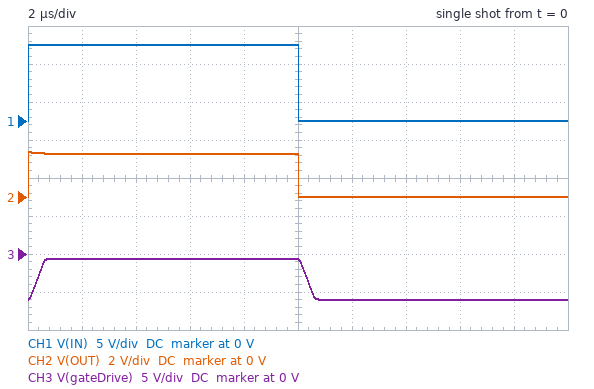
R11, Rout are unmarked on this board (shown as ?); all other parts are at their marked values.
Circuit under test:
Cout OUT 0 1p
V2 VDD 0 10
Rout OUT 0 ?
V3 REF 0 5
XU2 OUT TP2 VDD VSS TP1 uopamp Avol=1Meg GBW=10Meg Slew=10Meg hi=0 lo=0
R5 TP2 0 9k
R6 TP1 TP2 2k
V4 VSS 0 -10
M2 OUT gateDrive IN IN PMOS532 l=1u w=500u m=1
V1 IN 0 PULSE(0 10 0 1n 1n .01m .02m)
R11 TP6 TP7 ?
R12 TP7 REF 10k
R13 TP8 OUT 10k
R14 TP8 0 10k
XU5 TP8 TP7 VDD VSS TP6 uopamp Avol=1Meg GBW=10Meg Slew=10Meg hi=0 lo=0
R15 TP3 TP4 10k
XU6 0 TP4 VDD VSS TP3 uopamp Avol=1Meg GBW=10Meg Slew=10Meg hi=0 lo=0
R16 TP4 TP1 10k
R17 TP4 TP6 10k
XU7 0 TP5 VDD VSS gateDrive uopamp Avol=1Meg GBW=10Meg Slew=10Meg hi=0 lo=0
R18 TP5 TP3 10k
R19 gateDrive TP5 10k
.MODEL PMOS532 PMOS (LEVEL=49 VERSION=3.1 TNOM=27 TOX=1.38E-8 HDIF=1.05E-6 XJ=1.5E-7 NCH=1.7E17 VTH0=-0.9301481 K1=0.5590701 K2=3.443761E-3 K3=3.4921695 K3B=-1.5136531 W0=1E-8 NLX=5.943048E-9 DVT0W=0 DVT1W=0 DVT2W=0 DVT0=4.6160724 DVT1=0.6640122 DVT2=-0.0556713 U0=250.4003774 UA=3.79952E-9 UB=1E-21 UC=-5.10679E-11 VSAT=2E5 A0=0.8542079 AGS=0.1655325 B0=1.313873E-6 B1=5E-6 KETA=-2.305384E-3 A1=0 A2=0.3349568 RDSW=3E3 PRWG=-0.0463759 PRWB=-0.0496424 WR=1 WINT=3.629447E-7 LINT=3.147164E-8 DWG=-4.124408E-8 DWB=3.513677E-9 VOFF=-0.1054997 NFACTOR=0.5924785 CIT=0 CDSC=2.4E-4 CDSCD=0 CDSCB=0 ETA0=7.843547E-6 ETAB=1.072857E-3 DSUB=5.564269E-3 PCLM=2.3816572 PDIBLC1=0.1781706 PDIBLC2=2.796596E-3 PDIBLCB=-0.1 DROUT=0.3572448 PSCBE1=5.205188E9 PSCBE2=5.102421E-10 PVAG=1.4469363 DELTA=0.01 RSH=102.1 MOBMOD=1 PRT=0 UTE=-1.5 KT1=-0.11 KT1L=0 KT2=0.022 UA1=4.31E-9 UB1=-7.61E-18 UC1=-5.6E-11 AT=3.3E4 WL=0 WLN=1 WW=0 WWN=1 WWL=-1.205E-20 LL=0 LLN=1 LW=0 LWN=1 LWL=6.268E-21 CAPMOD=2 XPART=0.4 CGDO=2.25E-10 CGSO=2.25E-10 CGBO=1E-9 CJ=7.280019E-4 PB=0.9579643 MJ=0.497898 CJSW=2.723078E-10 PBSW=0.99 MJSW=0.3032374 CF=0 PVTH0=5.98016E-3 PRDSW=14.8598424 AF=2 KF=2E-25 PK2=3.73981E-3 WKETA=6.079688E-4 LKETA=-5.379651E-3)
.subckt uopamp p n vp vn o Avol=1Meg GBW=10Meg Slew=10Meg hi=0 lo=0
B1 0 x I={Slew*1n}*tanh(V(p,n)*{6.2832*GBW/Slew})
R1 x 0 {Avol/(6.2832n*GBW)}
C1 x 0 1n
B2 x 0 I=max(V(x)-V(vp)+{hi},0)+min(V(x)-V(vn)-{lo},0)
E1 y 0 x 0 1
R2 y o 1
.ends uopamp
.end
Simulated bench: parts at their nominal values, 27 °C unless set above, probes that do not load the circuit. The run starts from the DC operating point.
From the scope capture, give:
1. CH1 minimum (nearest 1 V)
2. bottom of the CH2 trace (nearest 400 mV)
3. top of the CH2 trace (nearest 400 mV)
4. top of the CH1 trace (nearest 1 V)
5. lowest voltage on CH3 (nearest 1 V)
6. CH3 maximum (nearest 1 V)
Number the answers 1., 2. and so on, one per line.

1. 0 V
2. 0 V
3. 2.4 V
4. 10 V
5. -6 V
6. -1 V
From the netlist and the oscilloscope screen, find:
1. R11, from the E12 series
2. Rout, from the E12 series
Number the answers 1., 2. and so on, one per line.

1. 12 kΩ
2. 68 Ω
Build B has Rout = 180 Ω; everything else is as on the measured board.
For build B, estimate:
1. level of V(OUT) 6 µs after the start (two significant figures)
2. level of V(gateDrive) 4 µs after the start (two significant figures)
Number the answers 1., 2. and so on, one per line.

1. 4.2 V
2. 3.7 V
